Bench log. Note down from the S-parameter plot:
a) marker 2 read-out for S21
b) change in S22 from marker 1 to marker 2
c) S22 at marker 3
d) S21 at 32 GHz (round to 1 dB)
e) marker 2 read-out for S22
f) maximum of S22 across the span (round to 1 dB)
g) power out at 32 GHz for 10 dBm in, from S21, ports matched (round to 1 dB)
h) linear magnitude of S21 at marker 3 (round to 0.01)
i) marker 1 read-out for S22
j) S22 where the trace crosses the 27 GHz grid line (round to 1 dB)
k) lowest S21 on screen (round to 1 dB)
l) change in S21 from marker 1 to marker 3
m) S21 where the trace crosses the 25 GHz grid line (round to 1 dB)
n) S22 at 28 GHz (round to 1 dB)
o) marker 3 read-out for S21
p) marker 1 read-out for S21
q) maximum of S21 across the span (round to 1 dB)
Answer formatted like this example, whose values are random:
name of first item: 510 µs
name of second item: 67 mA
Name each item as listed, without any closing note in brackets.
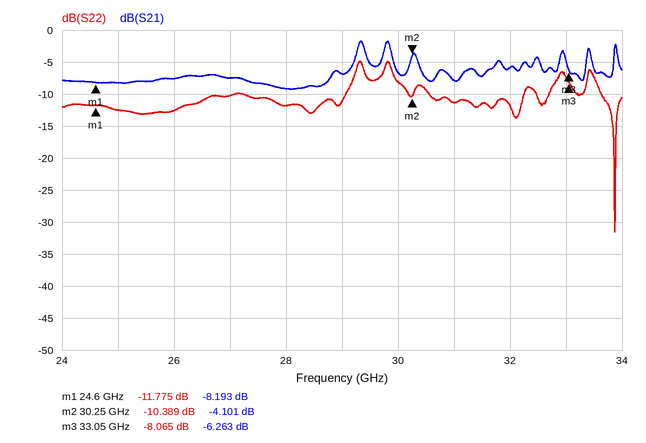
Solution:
marker 2 read-out for S21: -4.101 dB
change in S22 from marker 1 to marker 2: 1.386 dB
S22 at marker 3: -8.065 dB
S21 at 32 GHz: -6 dB
marker 2 read-out for S22: -10.389 dB
maximum of S22 across the span: -5 dB
power out at 32 GHz for 10 dBm in, from S21, ports matched: 4 dBm
linear magnitude of S21 at marker 3: 0.49
marker 1 read-out for S22: -11.775 dB
S22 where the trace crosses the 27 GHz grid line: -10 dB
lowest S21 on screen: -9 dB
change in S21 from marker 1 to marker 3: 1.930 dB
S21 where the trace crosses the 25 GHz grid line: -8 dB
S22 at 28 GHz: -12 dB
marker 3 read-out for S21: -6.263 dB
marker 1 read-out for S21: -8.193 dB
maximum of S21 across the span: -2 dB
